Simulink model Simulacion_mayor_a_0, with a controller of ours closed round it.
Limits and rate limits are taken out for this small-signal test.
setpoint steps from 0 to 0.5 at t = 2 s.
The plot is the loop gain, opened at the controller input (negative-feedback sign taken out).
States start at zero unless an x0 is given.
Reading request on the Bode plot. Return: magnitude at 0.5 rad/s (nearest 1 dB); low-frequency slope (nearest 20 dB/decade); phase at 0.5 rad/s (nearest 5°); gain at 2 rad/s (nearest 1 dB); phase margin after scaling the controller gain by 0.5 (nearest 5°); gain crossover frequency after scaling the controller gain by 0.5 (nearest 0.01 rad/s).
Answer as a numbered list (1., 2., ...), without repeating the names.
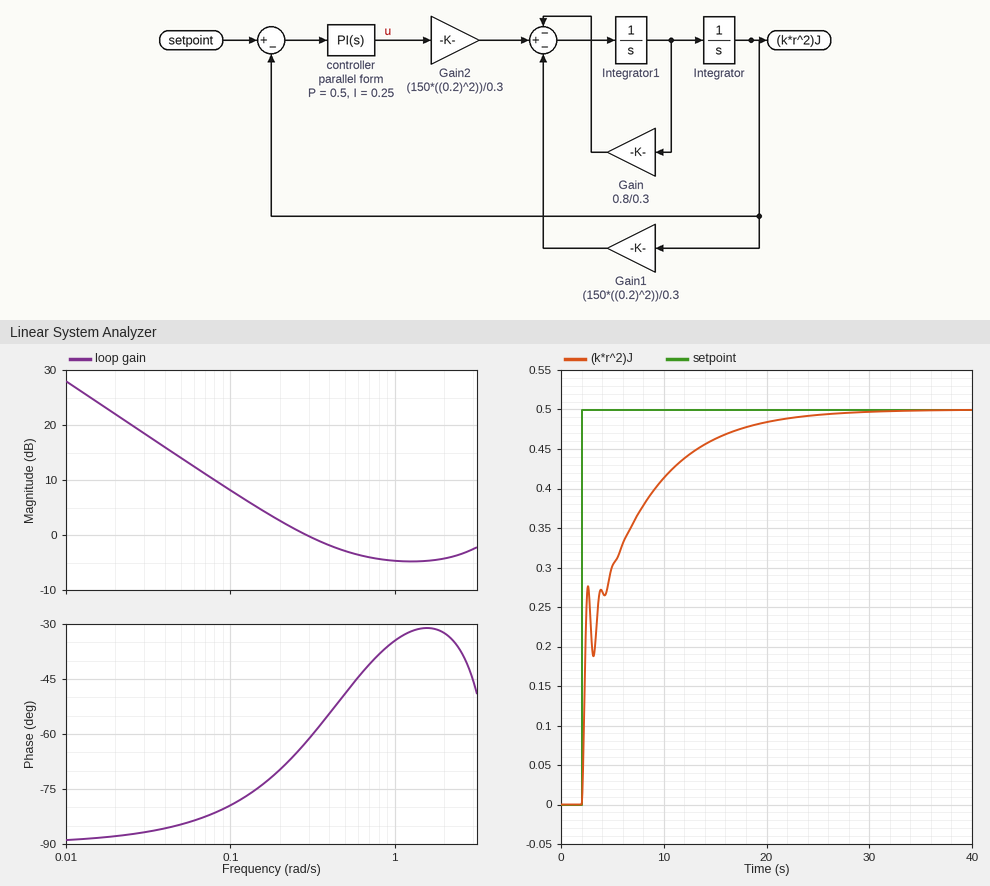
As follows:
1. -3 dB
2. -20 dB/decade
3. -50°
4. -4 dB
5. 105°
6. 0.13 rad/s
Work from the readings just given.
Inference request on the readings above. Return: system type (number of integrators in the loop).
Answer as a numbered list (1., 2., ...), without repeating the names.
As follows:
1. 1
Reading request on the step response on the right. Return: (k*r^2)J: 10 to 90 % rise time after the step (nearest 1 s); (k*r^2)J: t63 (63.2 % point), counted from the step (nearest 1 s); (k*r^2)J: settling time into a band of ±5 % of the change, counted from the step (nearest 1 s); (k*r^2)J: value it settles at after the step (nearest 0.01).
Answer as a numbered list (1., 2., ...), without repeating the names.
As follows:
1. 11 s
2. 4 s
3. 15 s
4. 0.50
